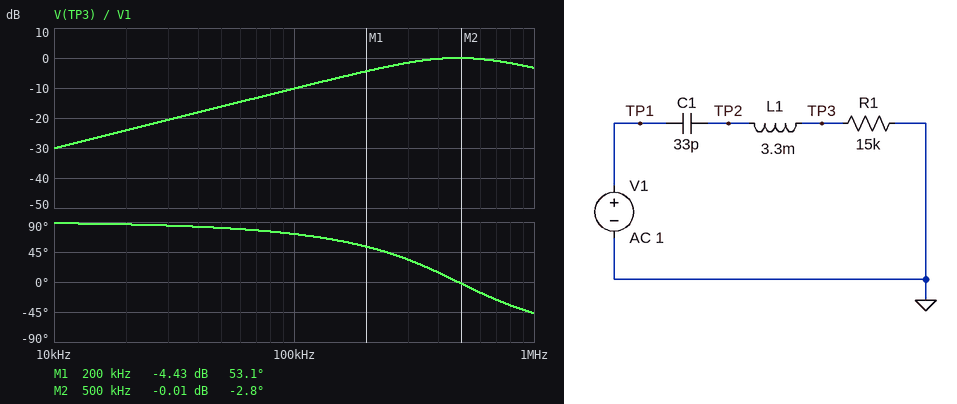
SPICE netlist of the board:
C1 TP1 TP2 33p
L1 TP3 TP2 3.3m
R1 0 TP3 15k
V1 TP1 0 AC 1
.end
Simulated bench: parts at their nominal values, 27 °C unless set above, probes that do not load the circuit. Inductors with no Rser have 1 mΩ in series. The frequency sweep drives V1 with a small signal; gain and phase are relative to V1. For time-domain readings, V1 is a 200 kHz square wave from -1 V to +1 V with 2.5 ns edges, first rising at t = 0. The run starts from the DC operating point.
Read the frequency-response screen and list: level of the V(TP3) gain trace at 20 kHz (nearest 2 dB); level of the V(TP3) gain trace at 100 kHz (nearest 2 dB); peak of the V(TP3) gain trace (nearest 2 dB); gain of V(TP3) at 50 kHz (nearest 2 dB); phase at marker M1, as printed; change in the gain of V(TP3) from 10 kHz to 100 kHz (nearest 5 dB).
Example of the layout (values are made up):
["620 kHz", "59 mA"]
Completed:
["-24 dB", "-10 dB", "0 dB", "-16 dB", "53.1 deg", "20 dB"]
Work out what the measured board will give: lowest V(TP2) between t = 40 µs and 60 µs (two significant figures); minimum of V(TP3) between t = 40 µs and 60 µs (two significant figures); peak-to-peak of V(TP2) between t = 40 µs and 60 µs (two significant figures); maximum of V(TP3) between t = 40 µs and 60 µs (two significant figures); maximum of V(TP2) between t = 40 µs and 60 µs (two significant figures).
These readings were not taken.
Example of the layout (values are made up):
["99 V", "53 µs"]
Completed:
["-2.0 V", "-1.3 V", "4.0 V", "1.3 V", "2.0 V"]
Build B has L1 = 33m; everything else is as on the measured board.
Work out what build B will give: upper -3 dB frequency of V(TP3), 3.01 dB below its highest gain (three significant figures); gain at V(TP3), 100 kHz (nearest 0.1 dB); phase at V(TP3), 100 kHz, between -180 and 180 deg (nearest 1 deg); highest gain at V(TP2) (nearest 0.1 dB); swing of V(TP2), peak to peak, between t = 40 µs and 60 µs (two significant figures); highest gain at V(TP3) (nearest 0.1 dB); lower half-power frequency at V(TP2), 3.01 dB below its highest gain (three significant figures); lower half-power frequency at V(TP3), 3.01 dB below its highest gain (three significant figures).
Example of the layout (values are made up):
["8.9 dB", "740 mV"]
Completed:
["193 kHz", "-6.4 dB", "61 deg", "7.5 dB", "4.7 V", "0 dB", "129 kHz", "121 kHz"]
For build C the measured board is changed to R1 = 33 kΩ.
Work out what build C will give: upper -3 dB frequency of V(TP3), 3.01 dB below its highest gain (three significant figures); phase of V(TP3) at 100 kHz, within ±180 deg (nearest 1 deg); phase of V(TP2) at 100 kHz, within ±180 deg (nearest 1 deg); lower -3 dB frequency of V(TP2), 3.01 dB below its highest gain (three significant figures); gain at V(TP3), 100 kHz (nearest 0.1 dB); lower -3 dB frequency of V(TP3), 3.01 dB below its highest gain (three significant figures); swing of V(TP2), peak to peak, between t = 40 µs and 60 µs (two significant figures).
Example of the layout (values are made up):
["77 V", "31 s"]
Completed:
["1.73 MHz", "54 deg", "58 deg", "150 kHz", "-4.7 dB", "135 kHz", "3.7 V"]
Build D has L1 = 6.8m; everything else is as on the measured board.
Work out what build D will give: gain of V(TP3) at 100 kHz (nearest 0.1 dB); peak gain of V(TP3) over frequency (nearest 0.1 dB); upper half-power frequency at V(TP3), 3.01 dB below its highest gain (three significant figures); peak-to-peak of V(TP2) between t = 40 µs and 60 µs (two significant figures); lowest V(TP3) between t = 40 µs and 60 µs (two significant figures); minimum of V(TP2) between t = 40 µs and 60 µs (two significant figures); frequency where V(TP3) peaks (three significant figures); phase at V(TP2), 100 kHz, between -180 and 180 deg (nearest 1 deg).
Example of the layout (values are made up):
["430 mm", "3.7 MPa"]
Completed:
["-9.8 dB", "0 dB", "555 kHz", "4.2 V", "-1.2 V", "-2.1 V", "336 kHz", "87 deg"]
